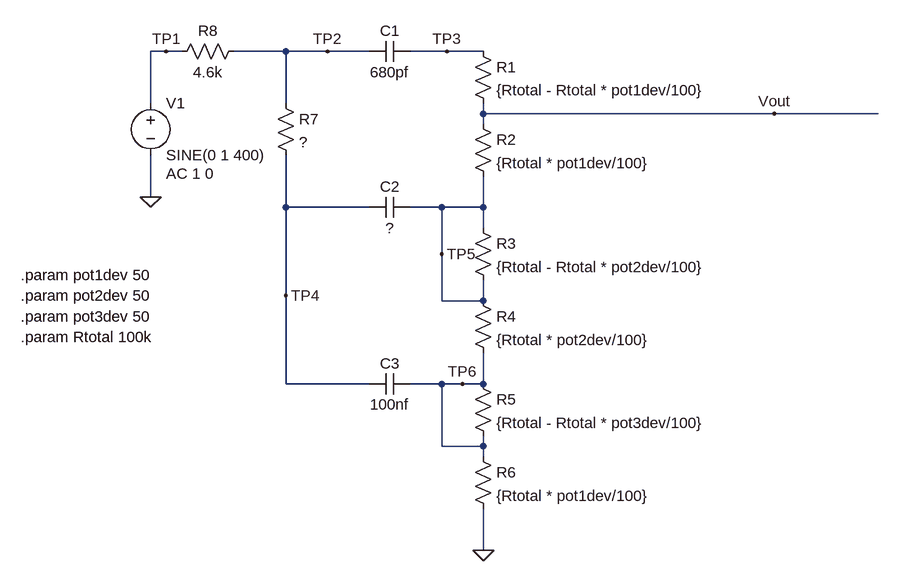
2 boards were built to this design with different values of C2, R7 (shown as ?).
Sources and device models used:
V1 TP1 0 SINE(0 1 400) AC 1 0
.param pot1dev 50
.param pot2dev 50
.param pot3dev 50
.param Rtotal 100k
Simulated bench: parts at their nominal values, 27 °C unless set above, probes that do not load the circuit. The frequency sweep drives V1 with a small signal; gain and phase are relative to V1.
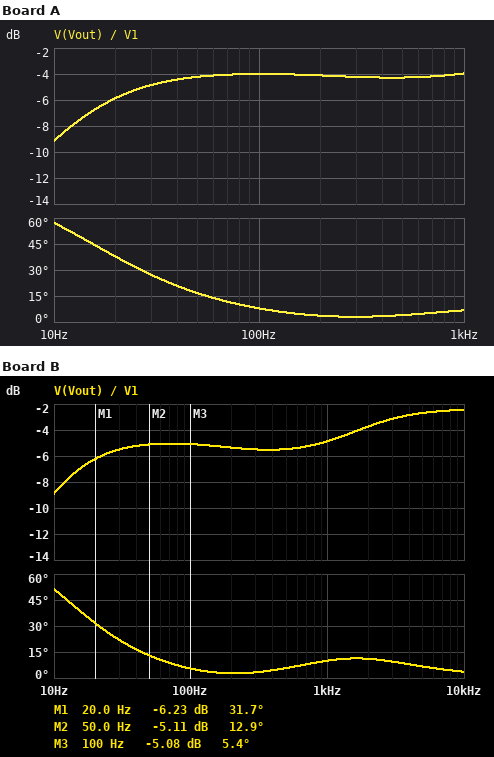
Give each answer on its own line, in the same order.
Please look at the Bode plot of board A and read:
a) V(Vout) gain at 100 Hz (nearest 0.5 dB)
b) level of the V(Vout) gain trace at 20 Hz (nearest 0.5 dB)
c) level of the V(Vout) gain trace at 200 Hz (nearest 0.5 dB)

-4.0 dB
-6.0 dB
-4.0 dB
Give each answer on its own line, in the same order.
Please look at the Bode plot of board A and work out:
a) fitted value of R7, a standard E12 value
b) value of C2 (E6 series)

33 kΩ
15 nF
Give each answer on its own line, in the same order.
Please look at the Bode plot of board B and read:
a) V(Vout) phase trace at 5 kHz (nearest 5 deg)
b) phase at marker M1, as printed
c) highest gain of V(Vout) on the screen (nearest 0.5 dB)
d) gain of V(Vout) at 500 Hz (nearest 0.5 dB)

5 deg
31.7 deg
-2.5 dB
-5.5 dB
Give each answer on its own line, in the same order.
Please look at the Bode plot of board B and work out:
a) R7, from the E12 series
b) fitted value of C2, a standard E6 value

47 kΩ
22 nF
